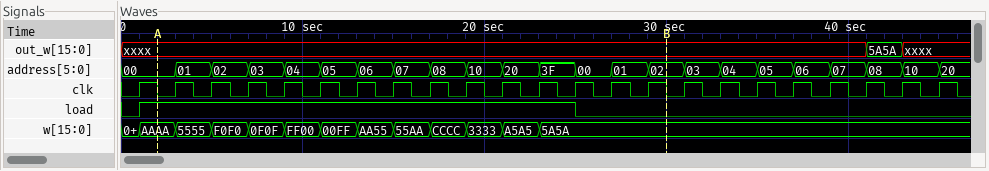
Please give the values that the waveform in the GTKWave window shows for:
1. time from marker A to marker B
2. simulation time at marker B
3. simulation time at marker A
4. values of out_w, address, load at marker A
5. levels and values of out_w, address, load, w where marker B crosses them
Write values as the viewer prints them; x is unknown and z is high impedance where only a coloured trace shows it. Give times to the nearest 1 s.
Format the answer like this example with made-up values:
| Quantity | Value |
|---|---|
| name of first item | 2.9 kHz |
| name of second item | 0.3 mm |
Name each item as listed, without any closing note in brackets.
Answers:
| Quantity | Value |
|---|---|
| time from marker A to marker B | 28 s |
| simulation time at marker B | 30 s |
| simulation time at marker A | 2 s |
| values of out_w, address, load at marker A | out_w=xxxx, address=00, load=1 |
| levels and values of out_w, address, load, w where marker B crosses them | out_w=xxxx, address=02, load=0, w=5A5A |
